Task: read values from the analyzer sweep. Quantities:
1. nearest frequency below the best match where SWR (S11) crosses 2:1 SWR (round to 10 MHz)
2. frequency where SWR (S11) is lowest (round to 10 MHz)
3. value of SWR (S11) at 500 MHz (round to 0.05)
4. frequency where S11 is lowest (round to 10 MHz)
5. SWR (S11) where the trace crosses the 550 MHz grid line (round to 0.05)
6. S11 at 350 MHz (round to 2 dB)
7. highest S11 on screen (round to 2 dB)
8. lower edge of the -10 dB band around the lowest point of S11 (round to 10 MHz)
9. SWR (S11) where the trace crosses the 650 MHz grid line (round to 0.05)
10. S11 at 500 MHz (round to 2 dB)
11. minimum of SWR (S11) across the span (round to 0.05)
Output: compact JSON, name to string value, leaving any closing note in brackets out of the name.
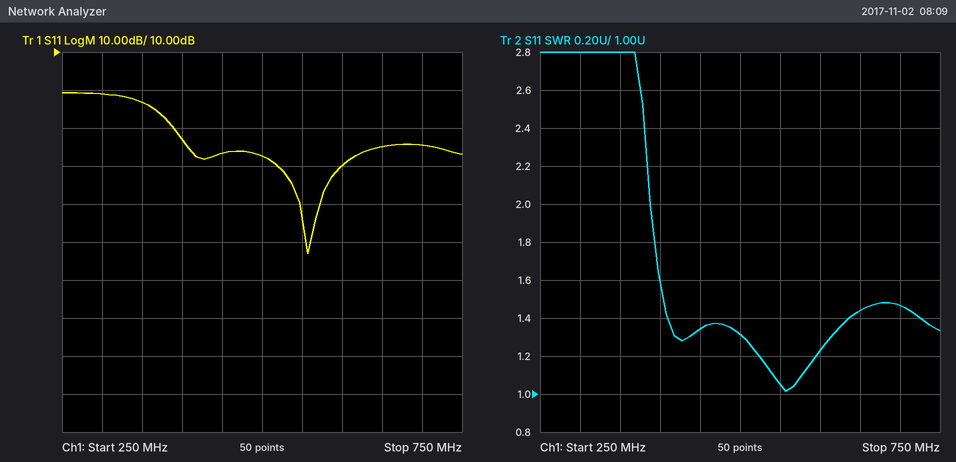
{"nearest frequency below the best match where SWR (S11) crosses 2:1 SWR": "390 MHz", "frequency where SWR (S11) is lowest": "560 MHz", "value of SWR (S11) at 500 MHz": "1.30", "frequency where S11 is lowest": "560 MHz", "SWR (S11) where the trace crosses the 550 MHz grid line": "1.05", "S11 at 350 MHz": "-4 dB", "highest S11 on screen": "0 dB", "lower edge of the -10 dB band around the lowest point of S11": "390 MHz", "SWR (S11) where the trace crosses the 650 MHz grid line": "1.45", "S11 at 500 MHz": "-18 dB", "minimum of SWR (S11) across the span": "1.00"}
